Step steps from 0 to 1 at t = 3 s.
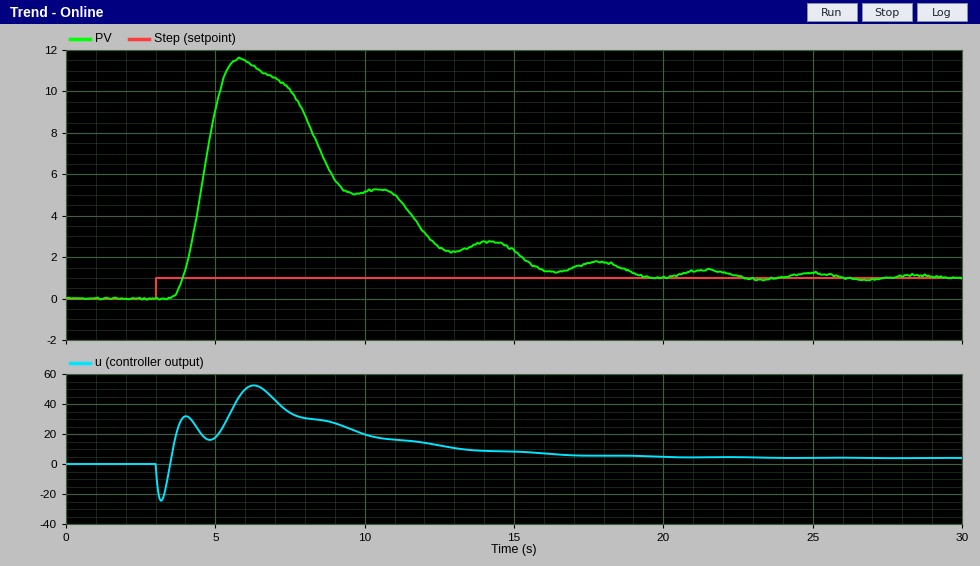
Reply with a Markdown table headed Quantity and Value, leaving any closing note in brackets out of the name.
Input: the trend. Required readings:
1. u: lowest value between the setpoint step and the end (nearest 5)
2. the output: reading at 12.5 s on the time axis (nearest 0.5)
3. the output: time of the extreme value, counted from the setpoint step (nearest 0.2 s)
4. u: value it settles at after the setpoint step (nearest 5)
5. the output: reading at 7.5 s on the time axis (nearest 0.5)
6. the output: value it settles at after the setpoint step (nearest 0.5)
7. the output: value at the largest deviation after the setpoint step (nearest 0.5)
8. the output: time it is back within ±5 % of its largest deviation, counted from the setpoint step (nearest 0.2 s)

| Quantity | Value |
|---|---|
| u: lowest value between the setpoint step and the end | -25 |
| the output: reading at 12.5 s on the time axis | 2.5 |
| the output: time of the extreme value, counted from the setpoint step | 2.8 s |
| u: value it settles at after the setpoint step | 5 |
| the output: reading at 7.5 s on the time axis | 10.0 |
| the output: value it settles at after the setpoint step | 1.0 |
| the output: value at the largest deviation after the setpoint step | 11.5 |
| the output: time it is back within ±5 % of its largest deviation, counted from the setpoint step | 15.4 s |
